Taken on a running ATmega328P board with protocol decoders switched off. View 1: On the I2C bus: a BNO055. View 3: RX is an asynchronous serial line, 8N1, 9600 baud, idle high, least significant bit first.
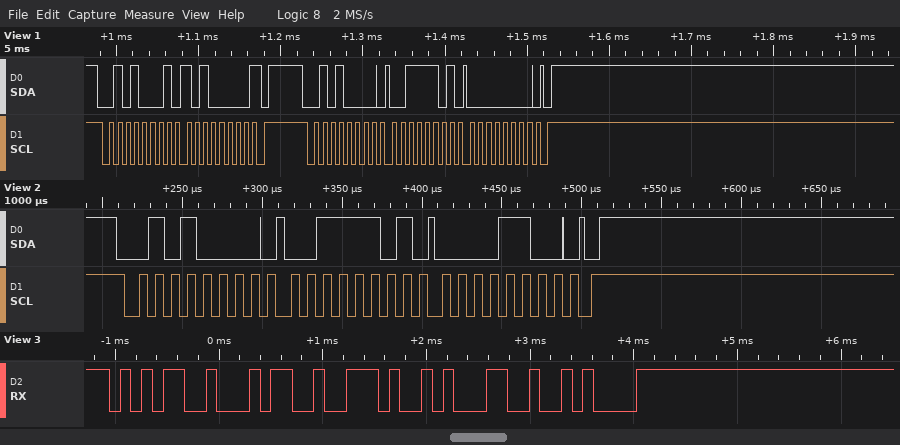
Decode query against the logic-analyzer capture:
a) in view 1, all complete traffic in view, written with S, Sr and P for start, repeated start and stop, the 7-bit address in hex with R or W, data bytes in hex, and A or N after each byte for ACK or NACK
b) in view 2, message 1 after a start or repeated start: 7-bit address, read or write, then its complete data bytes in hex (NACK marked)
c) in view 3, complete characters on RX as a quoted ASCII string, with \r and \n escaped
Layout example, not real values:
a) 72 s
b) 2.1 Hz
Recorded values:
a) S 28R A A0 N P S 28W A 3D A 00 A P
b) 0x28 write: 3D 0C
c) "54.1\n"
